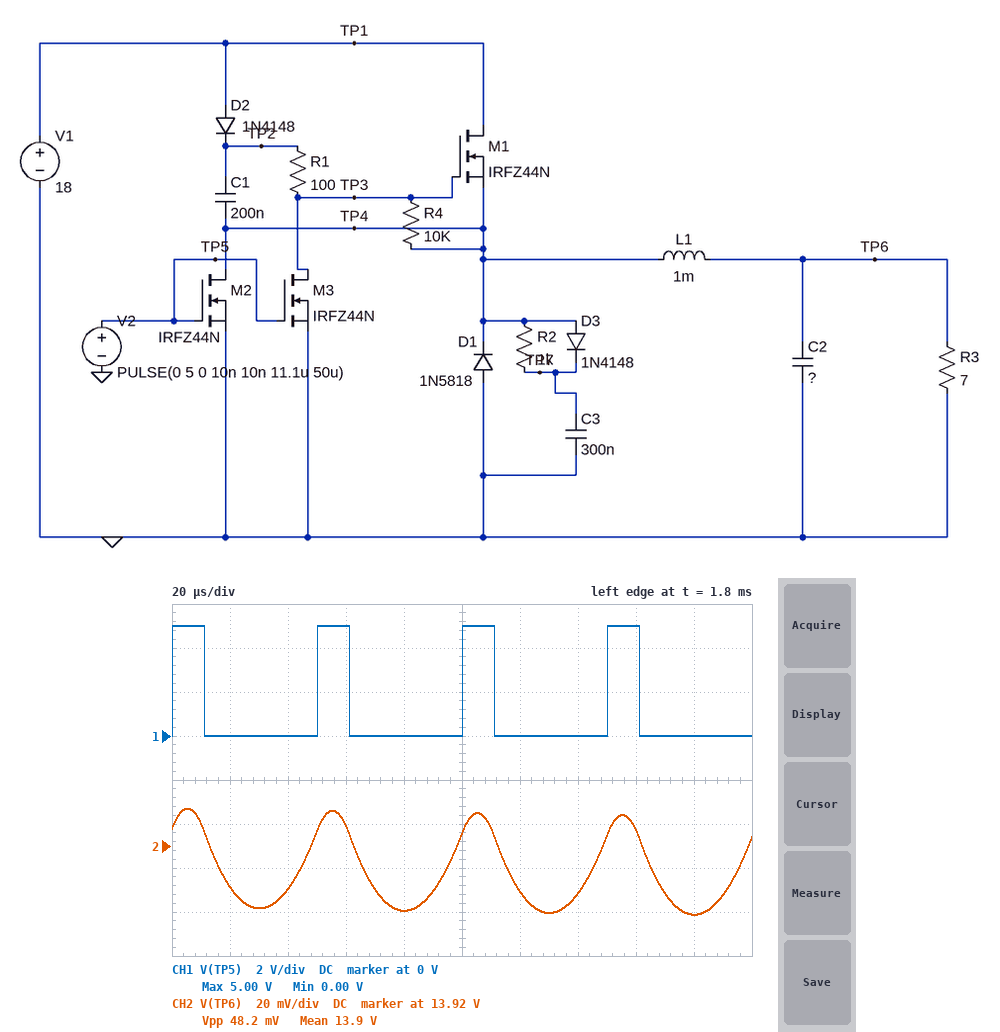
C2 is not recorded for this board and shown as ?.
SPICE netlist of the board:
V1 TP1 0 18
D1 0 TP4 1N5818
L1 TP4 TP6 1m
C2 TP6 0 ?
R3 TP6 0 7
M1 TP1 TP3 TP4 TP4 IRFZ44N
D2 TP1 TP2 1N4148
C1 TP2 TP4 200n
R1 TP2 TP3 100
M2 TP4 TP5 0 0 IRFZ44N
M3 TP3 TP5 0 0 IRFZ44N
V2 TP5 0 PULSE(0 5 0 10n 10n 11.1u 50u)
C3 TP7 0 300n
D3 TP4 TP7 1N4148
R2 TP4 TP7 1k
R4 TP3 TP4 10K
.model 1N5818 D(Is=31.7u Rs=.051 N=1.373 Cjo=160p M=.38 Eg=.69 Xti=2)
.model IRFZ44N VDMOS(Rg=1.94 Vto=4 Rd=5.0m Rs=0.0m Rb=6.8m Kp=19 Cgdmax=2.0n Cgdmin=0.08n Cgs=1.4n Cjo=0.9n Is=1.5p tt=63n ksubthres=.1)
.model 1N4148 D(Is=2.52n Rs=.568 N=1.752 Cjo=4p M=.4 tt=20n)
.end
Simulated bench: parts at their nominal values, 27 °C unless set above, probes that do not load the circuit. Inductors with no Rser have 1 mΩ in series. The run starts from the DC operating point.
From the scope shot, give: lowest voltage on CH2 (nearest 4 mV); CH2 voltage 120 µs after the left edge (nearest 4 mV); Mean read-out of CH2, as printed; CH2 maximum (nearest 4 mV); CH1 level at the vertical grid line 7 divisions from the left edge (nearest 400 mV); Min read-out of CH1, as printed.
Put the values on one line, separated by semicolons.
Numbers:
13.888 V; 13.900 V; 13.9 V; 13.936 V; 0 V; 0.00 V
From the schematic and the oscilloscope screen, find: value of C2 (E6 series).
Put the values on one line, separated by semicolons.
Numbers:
22 µF
